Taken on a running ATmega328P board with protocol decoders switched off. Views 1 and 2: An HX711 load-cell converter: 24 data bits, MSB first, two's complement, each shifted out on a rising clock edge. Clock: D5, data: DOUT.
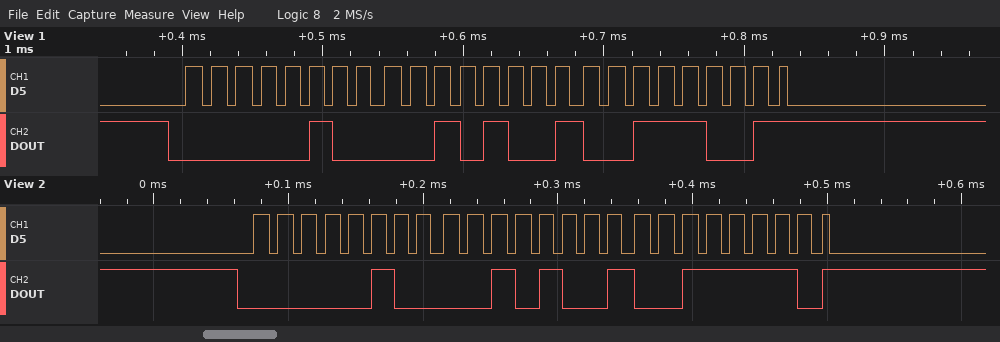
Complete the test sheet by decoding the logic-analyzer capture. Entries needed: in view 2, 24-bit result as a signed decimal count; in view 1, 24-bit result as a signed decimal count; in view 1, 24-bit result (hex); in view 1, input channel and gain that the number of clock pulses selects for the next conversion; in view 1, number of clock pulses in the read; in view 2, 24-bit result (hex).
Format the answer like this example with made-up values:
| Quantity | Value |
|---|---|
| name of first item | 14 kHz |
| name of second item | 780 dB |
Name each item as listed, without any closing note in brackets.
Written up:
| Quantity | Value |
|---|---|
| in view 2, 24-bit result as a signed decimal count | 272702 |
| in view 1, 24-bit result as a signed decimal count | 272697 |
| in view 1, 24-bit result | 0x042939 |
| in view 1, input channel and gain that the number of clock pulses selects for the next conversion | channel A, gain 128 |
| in view 1, number of clock pulses in the read | 25 |
| in view 2, 24-bit result | 0x04293E |
